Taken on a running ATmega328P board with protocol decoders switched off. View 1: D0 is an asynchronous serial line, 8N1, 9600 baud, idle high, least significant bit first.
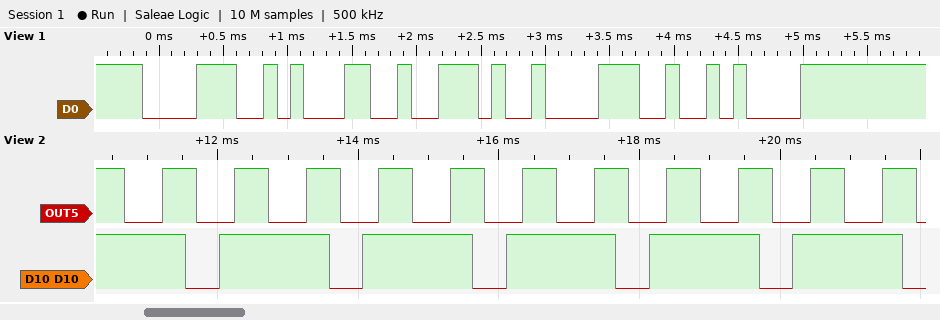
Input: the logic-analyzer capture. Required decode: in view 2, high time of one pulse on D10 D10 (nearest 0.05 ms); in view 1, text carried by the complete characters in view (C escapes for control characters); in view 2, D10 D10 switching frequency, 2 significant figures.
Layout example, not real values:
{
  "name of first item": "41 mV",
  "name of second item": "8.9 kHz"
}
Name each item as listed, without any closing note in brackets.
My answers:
{
  "in view 2, high time of one pulse on D10 D10": "1.55 ms",
  "in view 1, text carried by the complete characters in view": "\"81.8\\n\"",
  "in view 2, D10 D10 switching frequency, 2 significant figures": "490 Hz"
}
